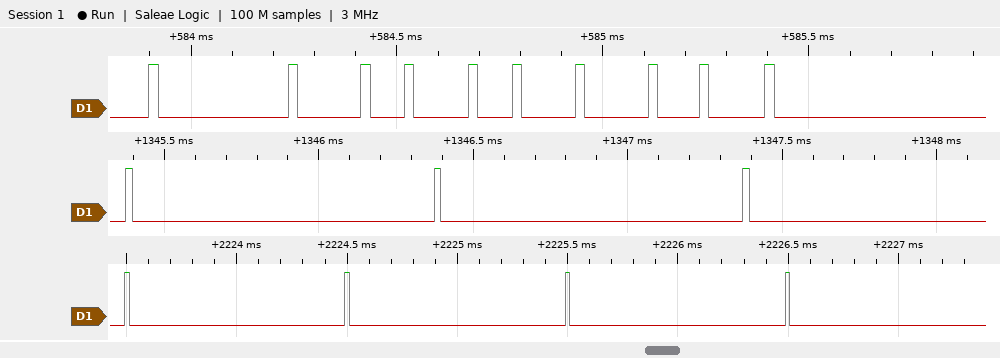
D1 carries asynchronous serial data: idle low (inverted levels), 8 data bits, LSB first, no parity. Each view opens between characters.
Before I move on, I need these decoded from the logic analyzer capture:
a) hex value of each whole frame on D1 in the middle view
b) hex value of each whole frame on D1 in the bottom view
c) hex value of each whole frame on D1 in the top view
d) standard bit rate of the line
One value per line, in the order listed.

FF, FF, FF
FF, FF, FF, FF
FF, BF, DF, DF, EF, FF
38400 baud
